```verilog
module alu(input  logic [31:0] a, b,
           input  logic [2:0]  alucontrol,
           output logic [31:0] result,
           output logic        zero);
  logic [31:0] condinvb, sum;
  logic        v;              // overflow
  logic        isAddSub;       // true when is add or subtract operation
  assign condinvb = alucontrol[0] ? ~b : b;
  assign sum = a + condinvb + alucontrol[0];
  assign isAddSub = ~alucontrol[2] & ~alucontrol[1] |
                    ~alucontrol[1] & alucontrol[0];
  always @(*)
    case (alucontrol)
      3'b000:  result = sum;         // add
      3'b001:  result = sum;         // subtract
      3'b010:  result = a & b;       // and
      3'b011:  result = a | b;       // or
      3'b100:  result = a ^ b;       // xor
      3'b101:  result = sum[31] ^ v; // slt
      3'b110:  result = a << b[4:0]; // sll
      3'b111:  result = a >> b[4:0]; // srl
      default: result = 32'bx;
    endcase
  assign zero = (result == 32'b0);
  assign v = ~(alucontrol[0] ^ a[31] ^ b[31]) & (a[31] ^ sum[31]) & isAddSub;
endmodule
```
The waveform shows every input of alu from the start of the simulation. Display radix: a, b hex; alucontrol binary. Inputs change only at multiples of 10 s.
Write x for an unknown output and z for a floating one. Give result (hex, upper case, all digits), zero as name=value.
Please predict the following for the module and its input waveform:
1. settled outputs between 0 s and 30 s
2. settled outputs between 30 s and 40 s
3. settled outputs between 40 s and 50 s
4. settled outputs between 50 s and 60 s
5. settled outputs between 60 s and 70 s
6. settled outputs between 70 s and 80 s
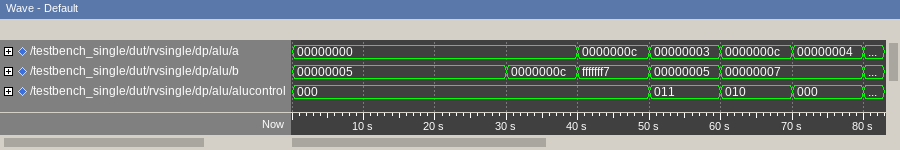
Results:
result=00000005, zero=0
result=0000000C, zero=0
result=00000003, zero=0
result=00000007, zero=0
result=00000004, zero=0
result=0000000B, zero=0
